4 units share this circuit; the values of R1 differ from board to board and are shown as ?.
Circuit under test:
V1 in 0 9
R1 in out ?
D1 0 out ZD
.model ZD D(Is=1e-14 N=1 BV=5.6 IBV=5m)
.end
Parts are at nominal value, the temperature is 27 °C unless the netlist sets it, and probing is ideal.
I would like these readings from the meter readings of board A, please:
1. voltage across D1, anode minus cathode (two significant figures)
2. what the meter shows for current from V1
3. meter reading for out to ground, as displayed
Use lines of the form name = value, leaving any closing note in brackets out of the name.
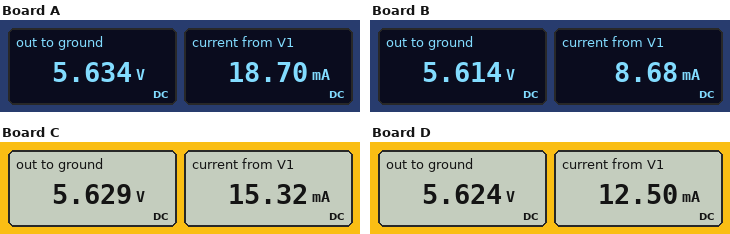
voltage across D1, anode minus cathode = -5.6 V
what the meter shows for current from V1 = 18.70 mA
meter reading for out to ground, as displayed = 5.634 V
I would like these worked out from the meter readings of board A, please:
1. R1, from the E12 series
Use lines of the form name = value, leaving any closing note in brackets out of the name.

R1, from the E12 series = 180 Ω
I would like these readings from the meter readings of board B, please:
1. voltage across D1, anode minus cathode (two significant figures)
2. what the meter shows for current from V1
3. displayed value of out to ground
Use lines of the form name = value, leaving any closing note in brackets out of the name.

voltage across D1, anode minus cathode = -5.6 V
what the meter shows for current from V1 = 8.68 mA
displayed value of out to ground = 5.614 V
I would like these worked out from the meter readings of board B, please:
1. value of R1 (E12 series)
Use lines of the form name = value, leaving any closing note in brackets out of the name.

value of R1 = 390 Ω
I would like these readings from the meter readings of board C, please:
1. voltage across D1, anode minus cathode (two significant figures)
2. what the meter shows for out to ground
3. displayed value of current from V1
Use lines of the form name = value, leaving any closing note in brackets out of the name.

voltage across D1, anode minus cathode = -5.6 V
what the meter shows for out to ground = 5.629 V
displayed value of current from V1 = 15.32 mA
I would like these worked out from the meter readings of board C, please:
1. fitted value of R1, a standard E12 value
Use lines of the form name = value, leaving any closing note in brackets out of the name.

fitted value of R1, a standard E12 value = 220 Ω
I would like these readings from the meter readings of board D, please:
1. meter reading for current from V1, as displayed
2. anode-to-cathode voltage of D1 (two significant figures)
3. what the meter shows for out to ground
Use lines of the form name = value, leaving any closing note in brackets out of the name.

meter reading for current from V1, as displayed = 12.50 mA
anode-to-cathode voltage of D1 = -5.6 V
what the meter shows for out to ground = 5.624 V
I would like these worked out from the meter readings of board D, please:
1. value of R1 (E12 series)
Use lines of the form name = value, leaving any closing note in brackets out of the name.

value of R1 = 270 Ω
